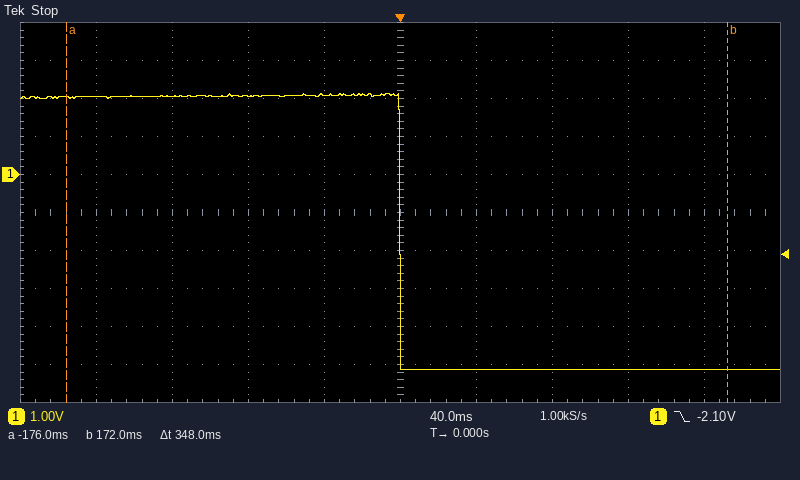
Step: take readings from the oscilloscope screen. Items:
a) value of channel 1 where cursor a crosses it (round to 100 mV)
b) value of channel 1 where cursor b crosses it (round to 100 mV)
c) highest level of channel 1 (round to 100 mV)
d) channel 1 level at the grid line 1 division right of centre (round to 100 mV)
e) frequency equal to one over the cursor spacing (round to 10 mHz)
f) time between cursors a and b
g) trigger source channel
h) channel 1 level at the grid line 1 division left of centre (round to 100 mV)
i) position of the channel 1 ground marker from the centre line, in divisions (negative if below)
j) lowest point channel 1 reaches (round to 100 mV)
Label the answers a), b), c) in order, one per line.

a) 2.0 V
b) -5.1 V
c) 2.1 V
d) -5.1 V
e) 2.87 Hz
f) 348 ms
g) channel 1
h) 2.1 V
i) +1.0 div
j) -5.1 V
